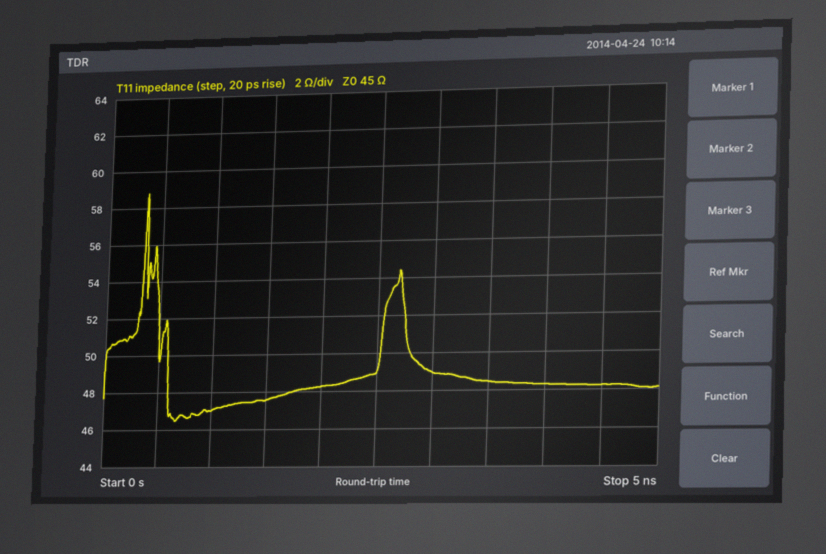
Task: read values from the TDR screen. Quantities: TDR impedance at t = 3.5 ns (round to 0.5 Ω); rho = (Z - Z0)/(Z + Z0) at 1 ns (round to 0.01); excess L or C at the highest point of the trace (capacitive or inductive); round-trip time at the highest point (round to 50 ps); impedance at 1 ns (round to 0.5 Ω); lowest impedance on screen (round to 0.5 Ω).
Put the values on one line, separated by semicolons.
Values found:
48.5 Ω; +0.02; inductive; 350 ps; 47.0 Ω; 46.5 Ω
